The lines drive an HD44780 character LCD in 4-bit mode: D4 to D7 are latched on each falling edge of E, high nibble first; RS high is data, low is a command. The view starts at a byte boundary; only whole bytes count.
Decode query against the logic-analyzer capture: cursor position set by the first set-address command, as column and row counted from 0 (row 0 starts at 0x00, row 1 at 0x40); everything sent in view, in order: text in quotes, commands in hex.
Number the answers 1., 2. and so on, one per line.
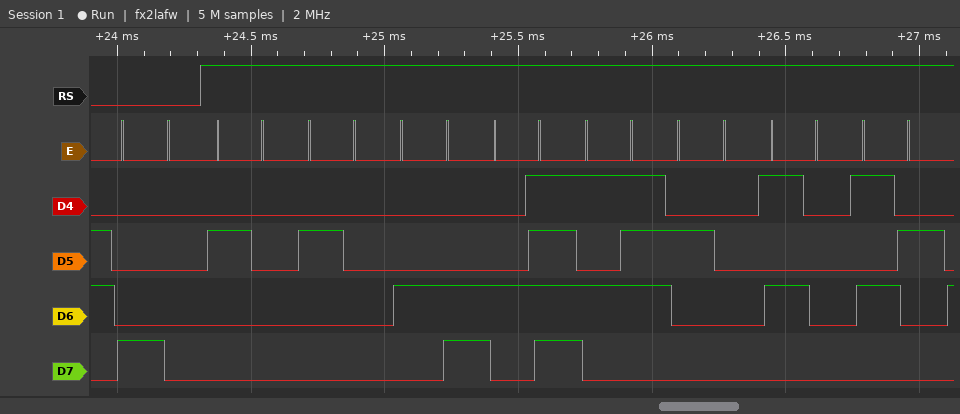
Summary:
1. column 0, row 0
2. 0x80 "  LOW PR"
